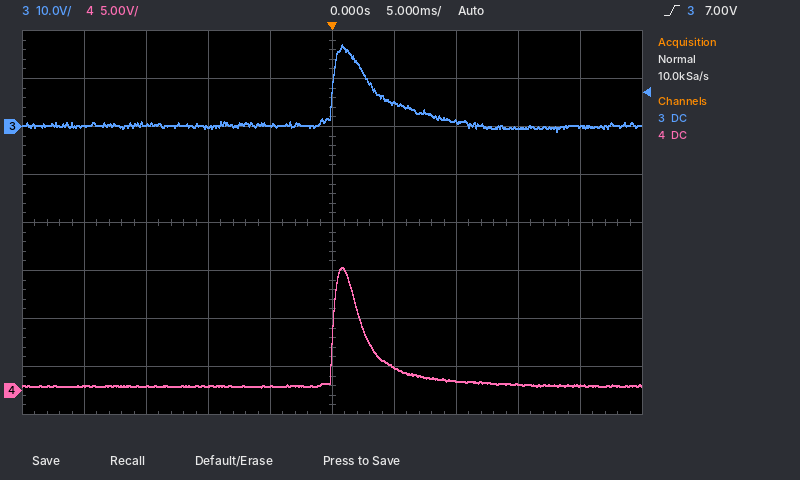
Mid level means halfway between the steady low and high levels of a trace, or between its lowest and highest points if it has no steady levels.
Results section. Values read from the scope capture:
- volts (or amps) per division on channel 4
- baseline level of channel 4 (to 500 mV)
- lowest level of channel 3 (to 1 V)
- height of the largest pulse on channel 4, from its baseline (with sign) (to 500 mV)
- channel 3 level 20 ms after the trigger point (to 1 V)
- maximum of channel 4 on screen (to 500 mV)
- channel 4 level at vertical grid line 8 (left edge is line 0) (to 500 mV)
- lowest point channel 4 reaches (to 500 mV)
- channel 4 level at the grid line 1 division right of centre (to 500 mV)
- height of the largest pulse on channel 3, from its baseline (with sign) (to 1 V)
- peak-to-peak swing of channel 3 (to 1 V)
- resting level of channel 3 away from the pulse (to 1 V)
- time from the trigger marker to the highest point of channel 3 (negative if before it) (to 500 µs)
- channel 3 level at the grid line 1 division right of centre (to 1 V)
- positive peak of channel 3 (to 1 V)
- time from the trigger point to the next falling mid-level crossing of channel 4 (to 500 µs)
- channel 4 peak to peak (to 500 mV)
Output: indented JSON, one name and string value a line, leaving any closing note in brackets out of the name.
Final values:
{
  "volts (or amps) per division on channel 4": "5 V",
  "baseline level of channel 4": "500 mV",
  "lowest level of channel 3": "-1 V",
  "height of the largest pulse on channel 4, from its baseline (with sign)": "+12.5 V",
  "channel 3 level 20 ms after the trigger point": "0 V",
  "maximum of channel 4 on screen": "13.0 V",
  "channel 4 level at vertical grid line 8 (left edge is line 0)": "500 mV",
  "lowest point channel 4 reaches": "500 mV",
  "channel 4 level at the grid line 1 division right of centre": "2.5 V",
  "height of the largest pulse on channel 3, from its baseline (with sign)": "+17 V",
  "peak-to-peak swing of channel 3": "18 V",
  "resting level of channel 3 away from the pulse": "0 V",
  "time from the trigger marker to the highest point of channel 3 (negative if before it)": "+1.0 ms",
  "channel 3 level at the grid line 1 division right of centre": "5 V",
  "positive peak of channel 3": "17 V",
  "time from the trigger point to the next falling mid-level crossing of channel 4": "2.5 ms",
  "channel 4 peak to peak": "12.5 V"
}
